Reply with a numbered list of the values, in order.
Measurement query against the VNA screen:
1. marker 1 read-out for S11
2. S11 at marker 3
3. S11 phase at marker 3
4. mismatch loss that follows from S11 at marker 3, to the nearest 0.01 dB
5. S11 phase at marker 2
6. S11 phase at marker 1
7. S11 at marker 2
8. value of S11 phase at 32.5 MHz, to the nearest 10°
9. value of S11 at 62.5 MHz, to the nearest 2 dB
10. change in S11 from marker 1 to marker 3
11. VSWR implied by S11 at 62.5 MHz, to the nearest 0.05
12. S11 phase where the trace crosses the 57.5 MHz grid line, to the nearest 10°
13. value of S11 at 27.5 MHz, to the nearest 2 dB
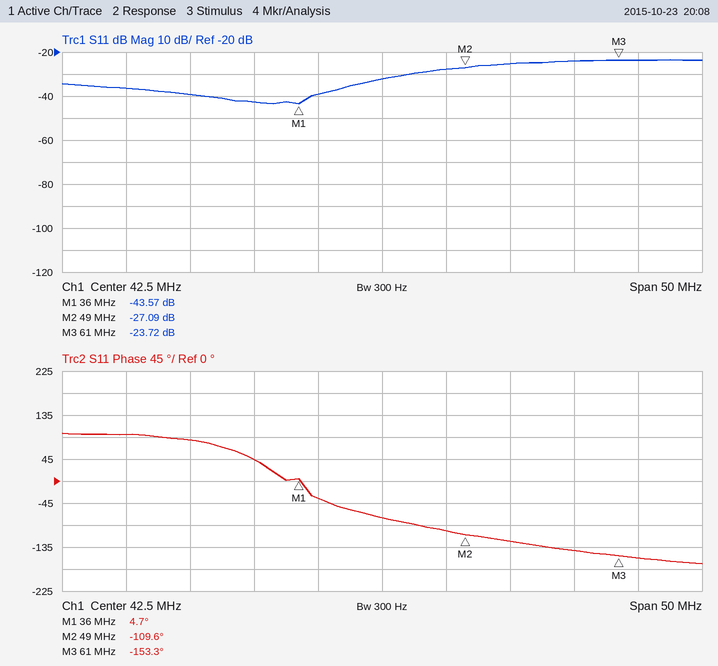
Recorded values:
1. -43.57 dB
2. -23.72 dB
3. -153.3°
4. 0.02 dB
5. -109.6°
6. 4.7°
7. -27.09 dB
8. 40°
9. -24 dB
10. 19.85 dB
11. 1.15
12. -140°
13. -40 dB
